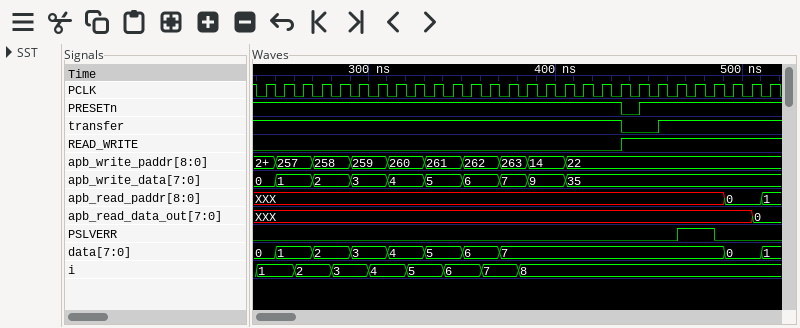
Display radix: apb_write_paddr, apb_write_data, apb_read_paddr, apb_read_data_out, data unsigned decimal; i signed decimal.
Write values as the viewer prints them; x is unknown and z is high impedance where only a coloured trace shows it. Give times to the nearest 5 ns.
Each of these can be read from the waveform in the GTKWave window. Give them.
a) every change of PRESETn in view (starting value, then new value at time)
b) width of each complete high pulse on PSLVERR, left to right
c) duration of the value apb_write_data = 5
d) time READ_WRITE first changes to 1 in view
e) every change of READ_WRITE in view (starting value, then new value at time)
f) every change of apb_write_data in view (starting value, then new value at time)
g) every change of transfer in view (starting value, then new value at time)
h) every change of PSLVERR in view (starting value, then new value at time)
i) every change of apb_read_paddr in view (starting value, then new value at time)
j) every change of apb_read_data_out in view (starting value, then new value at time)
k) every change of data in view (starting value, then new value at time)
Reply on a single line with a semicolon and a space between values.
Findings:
1, 0 at 435 ns, 1 at 445 ns; 20 ns; 20 ns; 435 ns; 0, 1 at 435 ns; 0, 1 at 250 ns, 2 at 270 ns, 3 at 290 ns, 4 at 310 ns, 5 at 330 ns, 6 at 350 ns, 7 at 370 ns, 9 at 385 ns, 35 at 405 ns; 1, 0 at 435 ns, 1 at 455 ns; 0, 1 at 465 ns, 0 at 485 ns; XXX, 0 at 490 ns, 1 at 510 ns; XXX, 0 at 505 ns; 0, 1 at 250 ns, 2 at 270 ns, 3 at 290 ns, 4 at 310 ns, 5 at 330 ns, 6 at 350 ns, 7 at 370 ns, 0 at 490 ns, 1 at 510 ns
